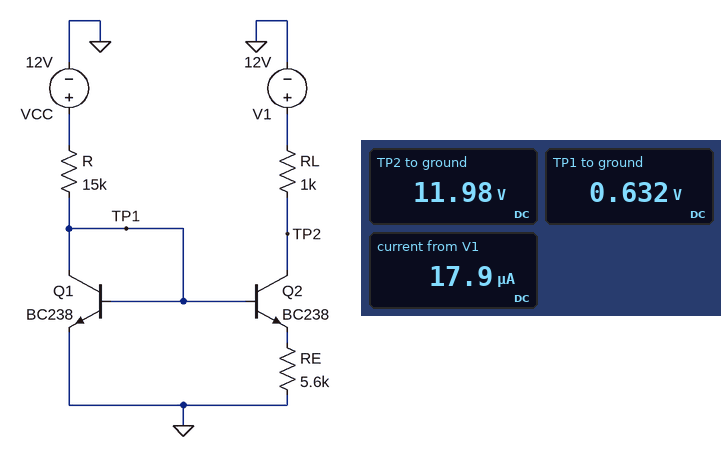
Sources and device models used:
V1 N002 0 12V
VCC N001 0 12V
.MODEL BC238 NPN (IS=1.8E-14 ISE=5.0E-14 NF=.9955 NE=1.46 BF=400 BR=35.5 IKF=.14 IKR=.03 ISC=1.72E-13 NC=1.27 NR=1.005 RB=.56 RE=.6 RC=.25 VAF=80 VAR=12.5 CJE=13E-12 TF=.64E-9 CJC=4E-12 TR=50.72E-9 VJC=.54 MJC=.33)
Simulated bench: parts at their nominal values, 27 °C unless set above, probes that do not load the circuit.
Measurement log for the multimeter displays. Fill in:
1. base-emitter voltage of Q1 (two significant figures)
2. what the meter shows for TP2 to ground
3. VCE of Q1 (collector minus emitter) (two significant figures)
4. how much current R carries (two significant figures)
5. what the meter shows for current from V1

630 mV
11.98 V
630 mV
760 µA
17.9 µA
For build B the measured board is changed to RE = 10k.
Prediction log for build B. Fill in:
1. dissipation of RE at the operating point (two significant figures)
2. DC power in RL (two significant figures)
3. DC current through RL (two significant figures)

1.3 µW
130 nW
11 µA
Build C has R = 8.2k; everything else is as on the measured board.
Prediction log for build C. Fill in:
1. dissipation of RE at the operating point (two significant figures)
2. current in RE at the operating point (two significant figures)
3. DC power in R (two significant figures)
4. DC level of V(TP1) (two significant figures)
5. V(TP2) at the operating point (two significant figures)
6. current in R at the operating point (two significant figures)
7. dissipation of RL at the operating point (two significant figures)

2.3 µW
20 µA
16 mW
650 mV
12 V
1.4 mA
410 nW
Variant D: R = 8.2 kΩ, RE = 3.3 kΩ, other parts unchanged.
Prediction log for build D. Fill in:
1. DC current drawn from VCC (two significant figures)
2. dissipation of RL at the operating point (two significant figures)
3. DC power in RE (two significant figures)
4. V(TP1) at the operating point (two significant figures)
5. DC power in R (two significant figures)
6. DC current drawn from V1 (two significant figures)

1.4 mA
960 nW
3.2 µW
650 mV
16 mW
31 µA
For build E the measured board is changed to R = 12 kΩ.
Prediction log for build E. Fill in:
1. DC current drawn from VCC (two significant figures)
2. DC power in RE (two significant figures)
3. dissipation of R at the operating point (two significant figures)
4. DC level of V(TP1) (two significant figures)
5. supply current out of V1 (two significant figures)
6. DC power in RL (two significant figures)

950 µA
2.0 µW
11 mW
640 mV
19 µA
350 nW
